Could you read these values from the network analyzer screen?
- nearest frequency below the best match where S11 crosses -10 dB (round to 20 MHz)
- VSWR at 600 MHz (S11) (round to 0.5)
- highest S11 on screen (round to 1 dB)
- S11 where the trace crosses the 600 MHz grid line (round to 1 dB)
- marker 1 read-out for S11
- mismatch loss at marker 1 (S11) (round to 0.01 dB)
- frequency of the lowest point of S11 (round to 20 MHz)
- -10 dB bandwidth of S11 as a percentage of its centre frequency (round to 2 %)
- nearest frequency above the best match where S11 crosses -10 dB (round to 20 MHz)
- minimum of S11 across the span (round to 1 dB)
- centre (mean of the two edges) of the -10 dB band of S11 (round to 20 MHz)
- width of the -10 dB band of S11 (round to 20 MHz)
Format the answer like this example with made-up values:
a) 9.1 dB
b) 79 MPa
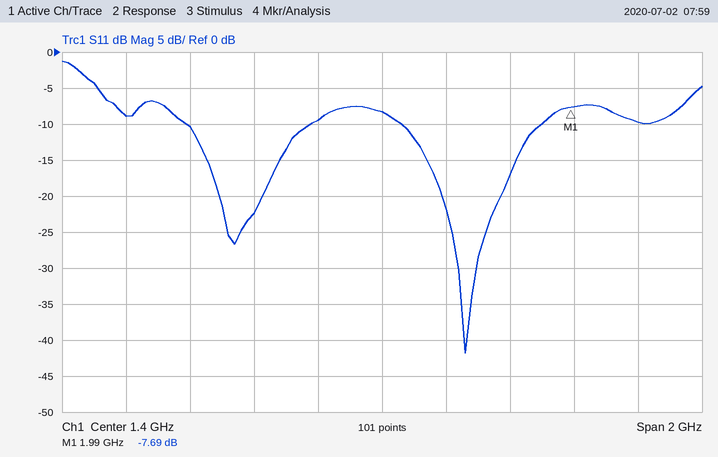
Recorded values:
a) 1.46 GHz
b) 2.0
c) -1 dB
d) -9 dB
e) -7.69 dB
f) 0.81 dB
g) 1.66 GHz
h) 26 %
i) 1.90 GHz
j) -42 dB
k) 1.68 GHz
l) 440 MHz
